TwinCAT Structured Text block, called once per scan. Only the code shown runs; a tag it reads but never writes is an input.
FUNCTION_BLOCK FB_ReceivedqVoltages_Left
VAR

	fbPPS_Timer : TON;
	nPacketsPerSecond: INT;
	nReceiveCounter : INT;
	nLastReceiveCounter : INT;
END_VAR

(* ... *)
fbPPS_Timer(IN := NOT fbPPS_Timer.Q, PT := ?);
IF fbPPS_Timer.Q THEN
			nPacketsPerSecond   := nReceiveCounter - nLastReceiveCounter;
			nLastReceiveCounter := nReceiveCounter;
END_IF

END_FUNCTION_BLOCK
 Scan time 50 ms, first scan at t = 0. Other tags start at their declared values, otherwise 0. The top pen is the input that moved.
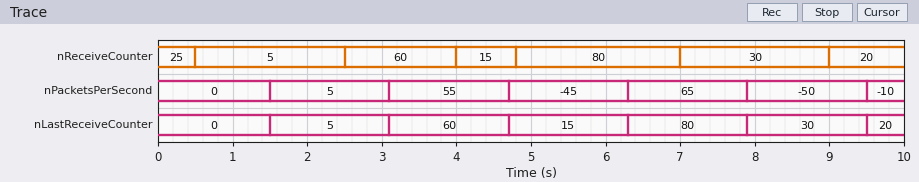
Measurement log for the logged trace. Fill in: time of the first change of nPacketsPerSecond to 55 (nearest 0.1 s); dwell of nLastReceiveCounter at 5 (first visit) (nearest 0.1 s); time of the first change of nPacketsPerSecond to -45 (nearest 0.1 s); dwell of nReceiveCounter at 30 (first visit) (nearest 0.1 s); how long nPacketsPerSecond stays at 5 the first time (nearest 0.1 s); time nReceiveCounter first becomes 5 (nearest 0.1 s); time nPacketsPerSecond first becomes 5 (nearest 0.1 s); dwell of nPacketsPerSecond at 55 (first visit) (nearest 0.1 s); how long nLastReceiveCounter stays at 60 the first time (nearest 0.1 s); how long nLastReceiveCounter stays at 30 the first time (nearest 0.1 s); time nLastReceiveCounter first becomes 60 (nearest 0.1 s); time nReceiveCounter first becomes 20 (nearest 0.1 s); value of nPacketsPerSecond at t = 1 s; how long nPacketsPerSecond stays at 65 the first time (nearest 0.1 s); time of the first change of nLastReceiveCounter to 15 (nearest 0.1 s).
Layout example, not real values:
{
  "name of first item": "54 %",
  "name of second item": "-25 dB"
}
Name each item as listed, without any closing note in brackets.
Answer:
{
  "time of the first change of nPacketsPerSecond to 55": "3.1 s",
  "dwell of nLastReceiveCounter at 5 (first visit)": "1.6 s",
  "time of the first change of nPacketsPerSecond to -45": "4.7 s",
  "dwell of nReceiveCounter at 30 (first visit)": "2.0 s",
  "how long nPacketsPerSecond stays at 5 the first time": "1.6 s",
  "time nReceiveCounter first becomes 5": "0.5 s",
  "time nPacketsPerSecond first becomes 5": "1.5 s",
  "dwell of nPacketsPerSecond at 55 (first visit)": "1.6 s",
  "how long nLastReceiveCounter stays at 60 the first time": "1.6 s",
  "how long nLastReceiveCounter stays at 30 the first time": "1.6 s",
  "time nLastReceiveCounter first becomes 60": "3.1 s",
  "time nReceiveCounter first becomes 20": "9.0 s",
  "value of nPacketsPerSecond at t = 1 s": "0",
  "how long nPacketsPerSecond stays at 65 the first time": "1.6 s",
  "time of the first change of nLastReceiveCounter to 15": "4.7 s"
}
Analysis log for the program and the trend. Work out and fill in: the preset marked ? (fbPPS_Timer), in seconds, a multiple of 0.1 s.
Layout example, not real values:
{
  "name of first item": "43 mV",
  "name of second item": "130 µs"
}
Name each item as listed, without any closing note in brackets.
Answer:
{
  "the preset marked ? (fbPPS_Timer), in seconds, a multiple of 0.1 s": "1.5 s"
}
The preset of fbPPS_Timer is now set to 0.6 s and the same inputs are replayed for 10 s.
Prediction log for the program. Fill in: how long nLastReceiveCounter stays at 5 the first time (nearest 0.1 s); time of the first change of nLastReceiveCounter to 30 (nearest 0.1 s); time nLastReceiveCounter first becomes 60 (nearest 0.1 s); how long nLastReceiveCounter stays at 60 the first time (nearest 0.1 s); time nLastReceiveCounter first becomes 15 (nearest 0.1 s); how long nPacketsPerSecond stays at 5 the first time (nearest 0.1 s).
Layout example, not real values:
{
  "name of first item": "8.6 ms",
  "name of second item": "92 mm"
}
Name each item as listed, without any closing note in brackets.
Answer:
{
  "how long nLastReceiveCounter stays at 5 the first time": "2.1 s",
  "time of the first change of nLastReceiveCounter to 30": "7.6 s",
  "time nLastReceiveCounter first becomes 60": "2.7 s",
  "how long nLastReceiveCounter stays at 60 the first time": "1.4 s",
  "time nLastReceiveCounter first becomes 15": "4.1 s",
  "how long nPacketsPerSecond stays at 5 the first time": "0.7 s"
}
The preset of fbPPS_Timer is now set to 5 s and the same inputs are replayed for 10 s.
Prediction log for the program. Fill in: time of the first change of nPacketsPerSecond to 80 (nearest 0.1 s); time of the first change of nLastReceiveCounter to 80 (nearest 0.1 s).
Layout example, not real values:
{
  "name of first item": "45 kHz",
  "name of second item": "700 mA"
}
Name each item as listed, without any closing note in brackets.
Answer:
{
  "time of the first change of nPacketsPerSecond to 80": "5.0 s",
  "time of the first change of nLastReceiveCounter to 80": "5.0 s"
}
